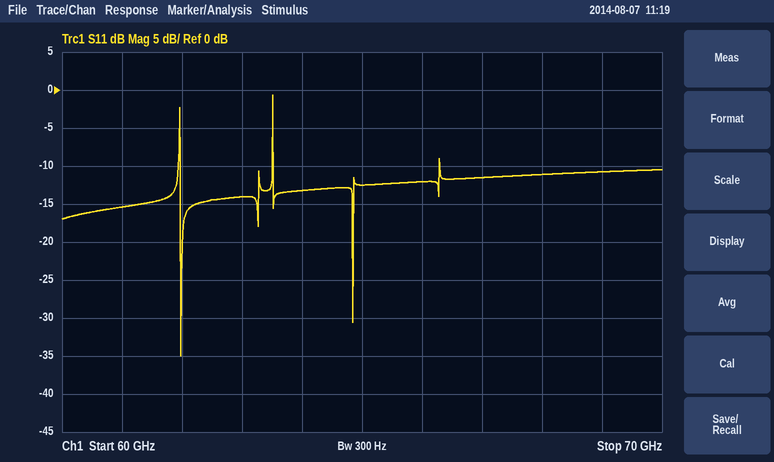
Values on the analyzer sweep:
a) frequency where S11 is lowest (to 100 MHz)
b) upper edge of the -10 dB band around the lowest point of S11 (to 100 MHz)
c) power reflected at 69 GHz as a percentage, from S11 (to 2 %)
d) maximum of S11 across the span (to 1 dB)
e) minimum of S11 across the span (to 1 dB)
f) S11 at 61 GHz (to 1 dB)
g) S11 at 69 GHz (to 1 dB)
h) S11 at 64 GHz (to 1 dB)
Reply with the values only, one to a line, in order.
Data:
62.0 GHz
63.5 GHz
8 %
-1 dB
-35 dB
-15 dB
-11 dB
-13 dB
